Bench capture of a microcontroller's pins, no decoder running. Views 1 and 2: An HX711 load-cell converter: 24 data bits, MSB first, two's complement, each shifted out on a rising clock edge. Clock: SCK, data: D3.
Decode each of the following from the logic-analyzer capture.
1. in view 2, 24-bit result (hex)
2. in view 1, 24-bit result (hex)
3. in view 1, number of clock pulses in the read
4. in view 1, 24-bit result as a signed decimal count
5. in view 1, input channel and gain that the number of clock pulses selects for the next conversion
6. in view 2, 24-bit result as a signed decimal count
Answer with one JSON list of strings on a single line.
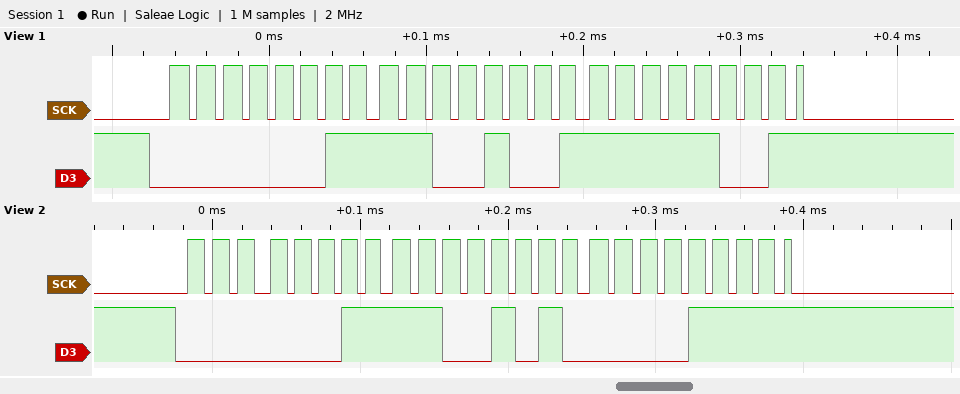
["0x03CA0F", "0x03C9F9", "25", "248313", "channel A, gain 128", "248335"]
